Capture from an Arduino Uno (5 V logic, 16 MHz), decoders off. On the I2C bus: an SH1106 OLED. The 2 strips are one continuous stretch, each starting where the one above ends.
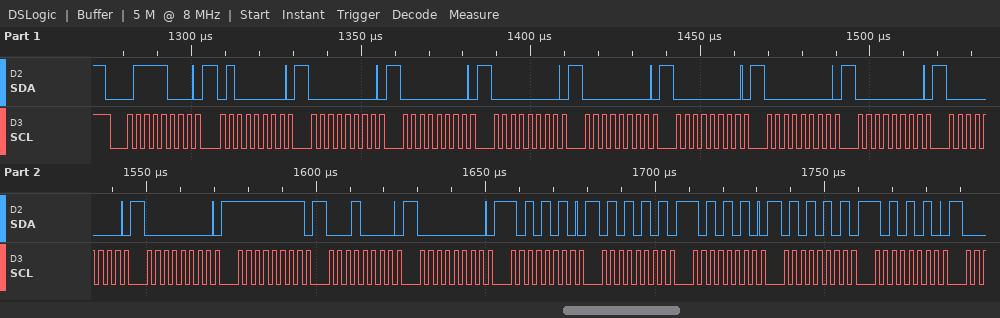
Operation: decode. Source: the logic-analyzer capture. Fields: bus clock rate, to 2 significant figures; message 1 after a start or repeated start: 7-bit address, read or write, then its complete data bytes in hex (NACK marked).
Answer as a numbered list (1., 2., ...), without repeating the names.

1. 400 kHz
2. 0x3C write: 40 00 00 00 00 00 00 00 00 00 FF 10 00 AA 55 AA 55 AA
